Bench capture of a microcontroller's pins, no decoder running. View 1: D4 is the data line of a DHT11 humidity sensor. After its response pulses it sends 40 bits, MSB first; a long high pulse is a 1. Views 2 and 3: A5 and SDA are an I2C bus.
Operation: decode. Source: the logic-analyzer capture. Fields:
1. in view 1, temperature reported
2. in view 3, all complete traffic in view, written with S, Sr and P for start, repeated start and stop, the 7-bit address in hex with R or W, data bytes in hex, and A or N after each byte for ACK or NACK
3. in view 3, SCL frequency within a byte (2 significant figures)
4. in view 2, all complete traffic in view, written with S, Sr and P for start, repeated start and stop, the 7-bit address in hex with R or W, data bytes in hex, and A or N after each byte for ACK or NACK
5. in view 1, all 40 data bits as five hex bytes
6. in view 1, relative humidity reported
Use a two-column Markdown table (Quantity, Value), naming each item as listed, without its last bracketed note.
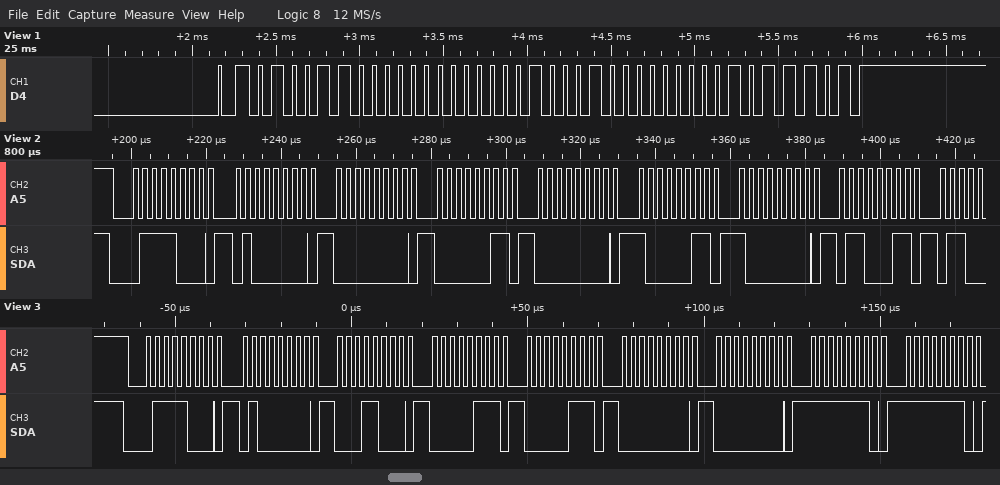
| Quantity | Value |
|---|---|
| in view 1, temperature reported | 17.0 °C |
| in view 3, all complete traffic in view, written with S, Sr and P for start, repeated start and stop, the 7-bit address in hex with R or W, data bytes in hex, and A or N after each byte for ACK or NACK | S 3CW A 40 A 18 A 07 A 07 A 00 A 00 A FE A FE A |
| in view 3, SCL frequency within a byte | 400 kHz |
| in view 2, all complete traffic in view, written with S, Sr and P for start, repeated start and stop, the 7-bit address in hex with R or W, data bytes in hex, and A or N after each byte for ACK or NACK | S 3CW A 40 A 00 A 03 A 00 A 83 A 80 A 63 A |
| in view 1, all 40 data bits as five hex bytes | 4C 00 11 00 5D |
| in view 1, relative humidity reported | 76 % |
